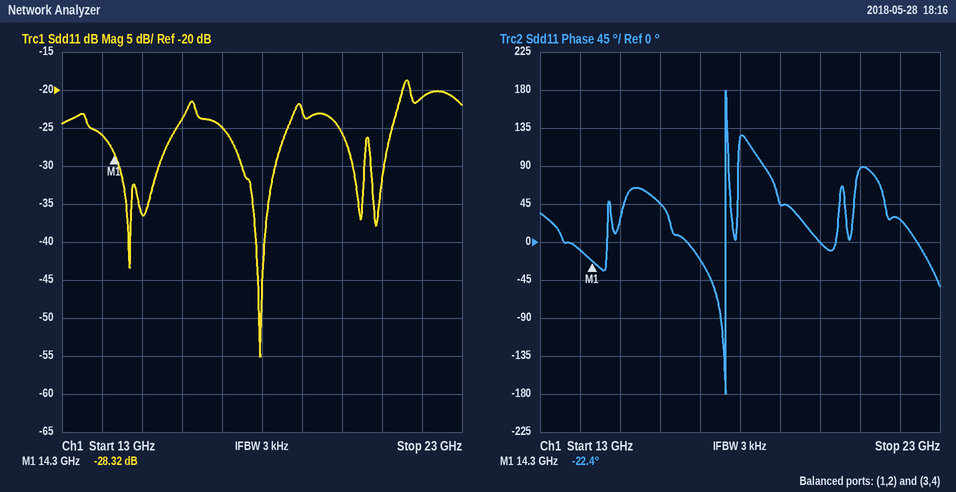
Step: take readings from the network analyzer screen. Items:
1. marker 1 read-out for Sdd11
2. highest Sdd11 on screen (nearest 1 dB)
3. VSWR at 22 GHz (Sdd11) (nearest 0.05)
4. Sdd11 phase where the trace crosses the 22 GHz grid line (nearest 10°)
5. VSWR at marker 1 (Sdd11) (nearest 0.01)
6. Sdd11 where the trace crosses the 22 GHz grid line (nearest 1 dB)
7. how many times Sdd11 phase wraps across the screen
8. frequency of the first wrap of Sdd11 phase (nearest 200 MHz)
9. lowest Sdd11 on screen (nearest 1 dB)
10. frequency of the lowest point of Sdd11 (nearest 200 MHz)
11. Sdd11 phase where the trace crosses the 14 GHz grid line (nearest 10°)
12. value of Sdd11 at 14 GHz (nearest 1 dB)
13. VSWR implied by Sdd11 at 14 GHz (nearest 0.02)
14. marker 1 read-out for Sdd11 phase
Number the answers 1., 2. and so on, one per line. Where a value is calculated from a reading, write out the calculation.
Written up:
1. -28.32 dB
2. -19 dB
3. |Γ| = 10^(-21/20) = 0.0891; VSWR = (1 + 0.0891)/(1 − 0.0891) ≈ 1.20
4. 30°
5. (1 + 0.0384)/(1 − 0.0384) ≈ 1.08
6. -21 dB
7. 1
8. 17.6 GHz
9. -55 dB
10. 18.0 GHz
11. -10°
12. -26 dB
13. |Γ| = 10^(-26/20) = 0.0501; VSWR = (1 + 0.0501)/(1 − 0.0501) ≈ 1.11, so 1.10 to the nearest 0.02
14. -22.4°
